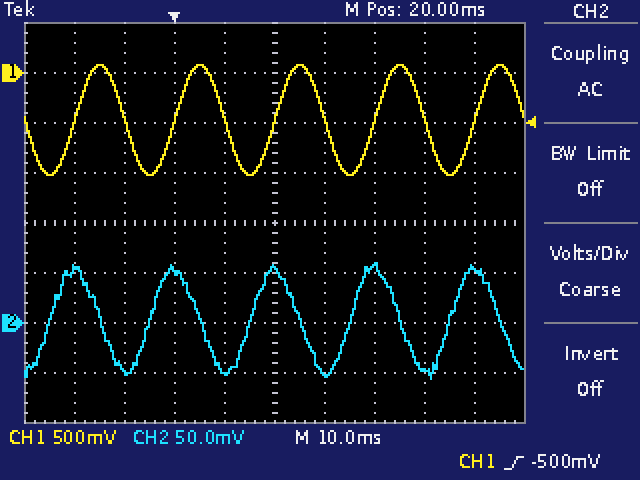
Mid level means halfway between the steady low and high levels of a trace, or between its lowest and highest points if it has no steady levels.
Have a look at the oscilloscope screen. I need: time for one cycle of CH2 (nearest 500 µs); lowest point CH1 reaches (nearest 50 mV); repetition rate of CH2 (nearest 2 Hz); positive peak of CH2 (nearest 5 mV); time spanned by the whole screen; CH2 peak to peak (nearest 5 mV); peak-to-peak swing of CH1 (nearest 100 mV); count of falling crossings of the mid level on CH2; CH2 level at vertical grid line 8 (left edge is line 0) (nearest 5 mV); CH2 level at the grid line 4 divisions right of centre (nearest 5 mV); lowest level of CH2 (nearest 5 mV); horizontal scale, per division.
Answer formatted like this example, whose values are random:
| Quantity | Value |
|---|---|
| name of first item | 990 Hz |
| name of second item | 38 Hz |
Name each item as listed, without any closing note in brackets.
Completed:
| Quantity | Value |
|---|---|
| time for one cycle of CH2 | 20.0 ms |
| lowest point CH1 reaches | -1.00 V |
| repetition rate of CH2 | 50 Hz |
| positive peak of CH2 | 60 mV |
| time spanned by the whole screen | 100 ms |
| CH2 peak to peak | 115 mV |
| peak-to-peak swing of CH1 | 1.10 V |
| count of falling crossings of the mid level on CH2 | 5 |
| CH2 level at vertical grid line 8 (left edge is line 0) | -45 mV |
| CH2 level at the grid line 4 divisions right of centre | 55 mV |
| lowest level of CH2 | -55 mV |
| horizontal scale, per division | 10 ms |
